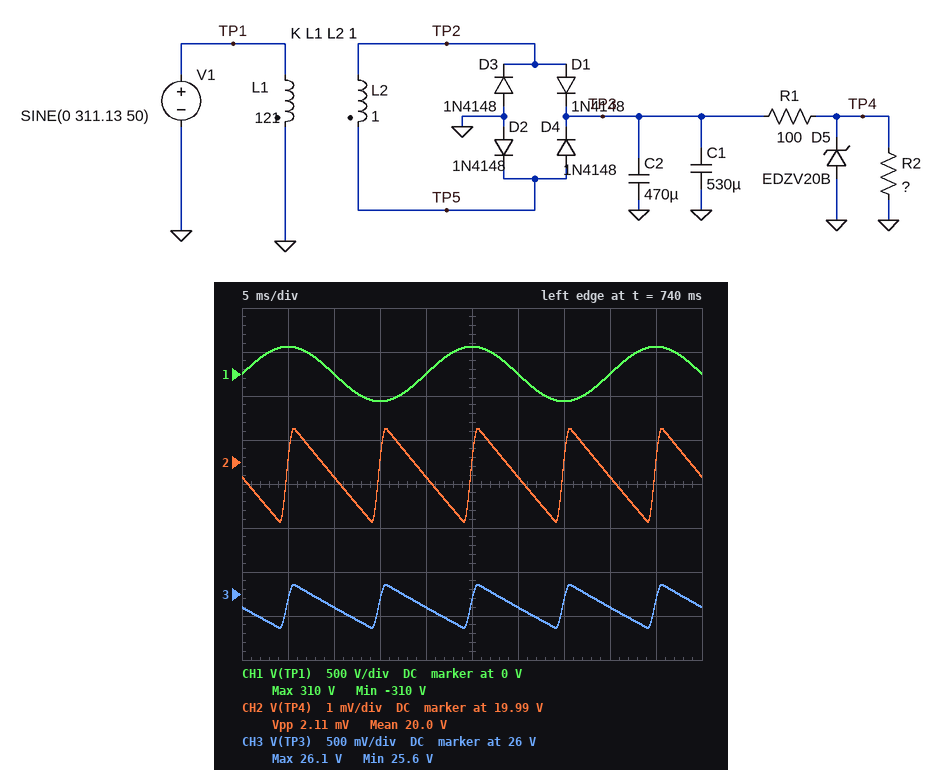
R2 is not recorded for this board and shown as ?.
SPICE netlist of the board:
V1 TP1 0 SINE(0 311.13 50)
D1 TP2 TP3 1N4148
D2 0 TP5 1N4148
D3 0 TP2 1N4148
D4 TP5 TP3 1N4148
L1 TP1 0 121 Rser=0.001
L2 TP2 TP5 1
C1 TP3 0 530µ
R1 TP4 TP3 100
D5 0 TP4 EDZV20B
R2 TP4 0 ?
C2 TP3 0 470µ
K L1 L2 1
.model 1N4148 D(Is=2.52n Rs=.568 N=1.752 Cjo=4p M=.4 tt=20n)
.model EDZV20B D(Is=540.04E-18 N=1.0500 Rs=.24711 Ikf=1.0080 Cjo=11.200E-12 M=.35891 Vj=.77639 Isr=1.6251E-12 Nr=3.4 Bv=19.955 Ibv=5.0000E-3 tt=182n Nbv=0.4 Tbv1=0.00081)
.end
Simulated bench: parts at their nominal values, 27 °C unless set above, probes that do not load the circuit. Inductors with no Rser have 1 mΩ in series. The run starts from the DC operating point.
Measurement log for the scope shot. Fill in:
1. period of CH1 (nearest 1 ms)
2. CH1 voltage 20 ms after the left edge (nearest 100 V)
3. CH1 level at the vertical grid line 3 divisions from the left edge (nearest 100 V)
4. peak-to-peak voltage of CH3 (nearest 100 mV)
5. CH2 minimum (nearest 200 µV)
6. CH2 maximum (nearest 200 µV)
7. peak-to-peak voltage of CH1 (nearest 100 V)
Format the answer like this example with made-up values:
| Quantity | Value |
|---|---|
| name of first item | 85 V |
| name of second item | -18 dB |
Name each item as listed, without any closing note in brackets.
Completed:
| Quantity | Value |
|---|---|
| period of CH1 | 20 ms |
| CH1 voltage 20 ms after the left edge | 0 V |
| CH1 level at the vertical grid line 3 divisions from the left edge | -300 V |
| peak-to-peak voltage of CH3 | 500 mV |
| CH2 minimum | 19.9926 V |
| CH2 maximum | 19.9948 V |
| peak-to-peak voltage of CH1 | 600 V |
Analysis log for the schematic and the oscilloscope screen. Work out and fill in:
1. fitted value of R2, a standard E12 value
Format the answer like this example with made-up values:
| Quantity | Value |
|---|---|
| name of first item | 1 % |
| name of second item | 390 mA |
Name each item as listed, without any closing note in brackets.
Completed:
| Quantity | Value |
|---|---|
| fitted value of R2, a standard E12 value | 6.8 kΩ |
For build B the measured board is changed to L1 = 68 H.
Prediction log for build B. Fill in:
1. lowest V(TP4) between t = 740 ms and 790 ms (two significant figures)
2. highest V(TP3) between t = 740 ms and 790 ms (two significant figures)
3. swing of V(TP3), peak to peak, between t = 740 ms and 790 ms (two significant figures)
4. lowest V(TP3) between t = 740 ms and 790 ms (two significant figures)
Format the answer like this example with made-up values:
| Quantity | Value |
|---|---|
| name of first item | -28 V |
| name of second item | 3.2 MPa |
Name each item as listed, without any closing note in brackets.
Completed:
| Quantity | Value |
|---|---|
| lowest V(TP4) between t = 740 ms and 790 ms | 20 V |
| highest V(TP3) between t = 740 ms and 790 ms | 35 V |
| swing of V(TP3), peak to peak, between t = 740 ms and 790 ms | 1.2 V |
| lowest V(TP3) between t = 740 ms and 790 ms | 34 V |
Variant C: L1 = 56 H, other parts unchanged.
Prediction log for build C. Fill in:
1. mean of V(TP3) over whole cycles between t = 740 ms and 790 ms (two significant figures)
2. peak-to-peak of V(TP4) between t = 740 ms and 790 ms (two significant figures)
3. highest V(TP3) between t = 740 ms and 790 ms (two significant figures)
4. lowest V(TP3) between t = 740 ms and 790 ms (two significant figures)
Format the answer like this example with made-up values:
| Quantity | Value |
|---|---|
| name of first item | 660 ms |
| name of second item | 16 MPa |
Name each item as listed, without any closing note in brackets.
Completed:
| Quantity | Value |
|---|---|
| mean of V(TP3) over whole cycles between t = 740 ms and 790 ms | 38 V |
| peak-to-peak of V(TP4) between t = 740 ms and 790 ms | 4.4 mV |
| highest V(TP3) between t = 740 ms and 790 ms | 39 V |
| lowest V(TP3) between t = 740 ms and 790 ms | 37 V |
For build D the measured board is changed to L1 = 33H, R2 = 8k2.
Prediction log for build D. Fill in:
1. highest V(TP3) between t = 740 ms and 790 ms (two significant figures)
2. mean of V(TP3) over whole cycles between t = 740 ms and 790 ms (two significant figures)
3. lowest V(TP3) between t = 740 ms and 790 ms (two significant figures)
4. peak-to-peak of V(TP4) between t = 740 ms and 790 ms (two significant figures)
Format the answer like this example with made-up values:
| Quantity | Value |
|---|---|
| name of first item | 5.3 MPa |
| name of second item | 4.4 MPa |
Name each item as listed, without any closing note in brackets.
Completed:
| Quantity | Value |
|---|---|
| highest V(TP3) between t = 740 ms and 790 ms | 51 V |
| mean of V(TP3) over whole cycles between t = 740 ms and 790 ms | 50 V |
| lowest V(TP3) between t = 740 ms and 790 ms | 48 V |
| peak-to-peak of V(TP4) between t = 740 ms and 790 ms | 6.6 mV |
